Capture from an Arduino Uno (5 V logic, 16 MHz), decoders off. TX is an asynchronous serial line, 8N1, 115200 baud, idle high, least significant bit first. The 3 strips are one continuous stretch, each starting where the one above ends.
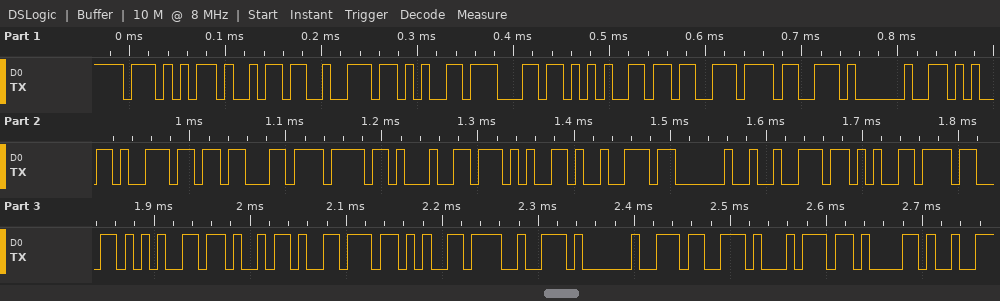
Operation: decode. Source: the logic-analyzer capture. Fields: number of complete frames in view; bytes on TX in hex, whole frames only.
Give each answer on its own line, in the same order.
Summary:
29
57 69 72 65 6C 65 73 73 20 65 6E 63 6F 64 65 72 20 72 65 63 65 69 76 65 72 20 73 74 61
